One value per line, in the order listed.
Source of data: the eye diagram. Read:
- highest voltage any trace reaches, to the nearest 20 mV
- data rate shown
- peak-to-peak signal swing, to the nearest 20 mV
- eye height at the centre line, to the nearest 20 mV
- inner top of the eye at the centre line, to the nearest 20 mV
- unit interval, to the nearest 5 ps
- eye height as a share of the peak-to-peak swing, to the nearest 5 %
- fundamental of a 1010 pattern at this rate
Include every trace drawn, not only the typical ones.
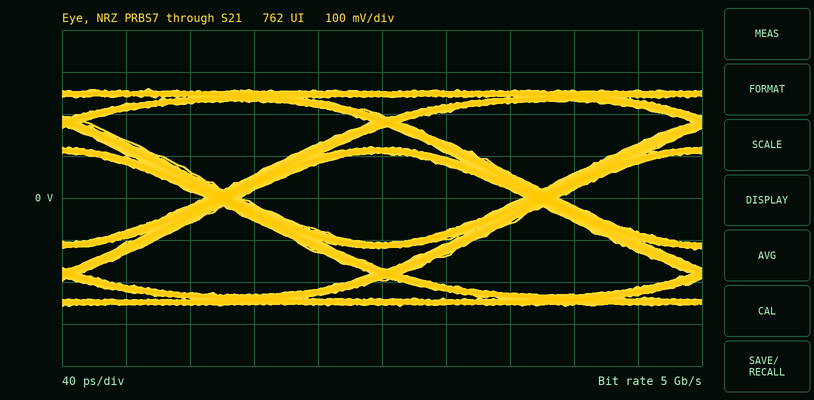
260 mV
5 Gb/s
520 mV
220 mV
100 mV
200 ps
40 %
2.5 GHz
